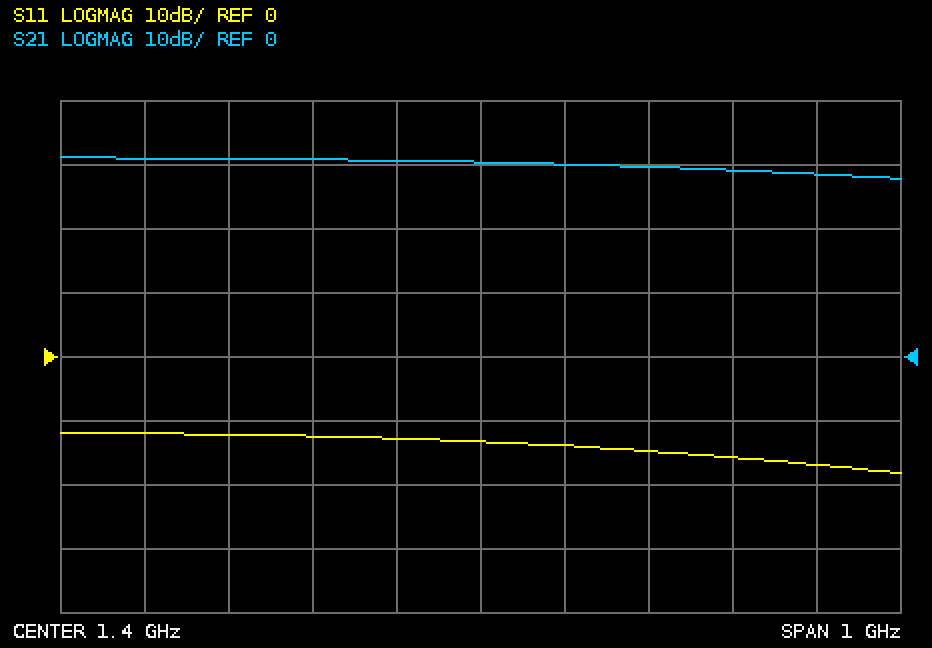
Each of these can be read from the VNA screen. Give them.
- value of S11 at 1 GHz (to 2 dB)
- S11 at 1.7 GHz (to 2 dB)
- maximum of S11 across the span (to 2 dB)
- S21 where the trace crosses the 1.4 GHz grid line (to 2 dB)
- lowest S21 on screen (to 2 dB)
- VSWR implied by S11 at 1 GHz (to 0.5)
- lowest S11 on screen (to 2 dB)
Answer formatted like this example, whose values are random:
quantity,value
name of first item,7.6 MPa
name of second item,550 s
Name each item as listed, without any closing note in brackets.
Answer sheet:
quantity,value
value of S11 at 1 GHz,-12 dB
S11 at 1.7 GHz,-16 dB
maximum of S11 across the span,-12 dB
S21 where the trace crosses the 1.4 GHz grid line,30 dB
lowest S21 on screen,28 dB
VSWR implied by S11 at 1 GHz,1.5
lowest S11 on screen,-18 dB
